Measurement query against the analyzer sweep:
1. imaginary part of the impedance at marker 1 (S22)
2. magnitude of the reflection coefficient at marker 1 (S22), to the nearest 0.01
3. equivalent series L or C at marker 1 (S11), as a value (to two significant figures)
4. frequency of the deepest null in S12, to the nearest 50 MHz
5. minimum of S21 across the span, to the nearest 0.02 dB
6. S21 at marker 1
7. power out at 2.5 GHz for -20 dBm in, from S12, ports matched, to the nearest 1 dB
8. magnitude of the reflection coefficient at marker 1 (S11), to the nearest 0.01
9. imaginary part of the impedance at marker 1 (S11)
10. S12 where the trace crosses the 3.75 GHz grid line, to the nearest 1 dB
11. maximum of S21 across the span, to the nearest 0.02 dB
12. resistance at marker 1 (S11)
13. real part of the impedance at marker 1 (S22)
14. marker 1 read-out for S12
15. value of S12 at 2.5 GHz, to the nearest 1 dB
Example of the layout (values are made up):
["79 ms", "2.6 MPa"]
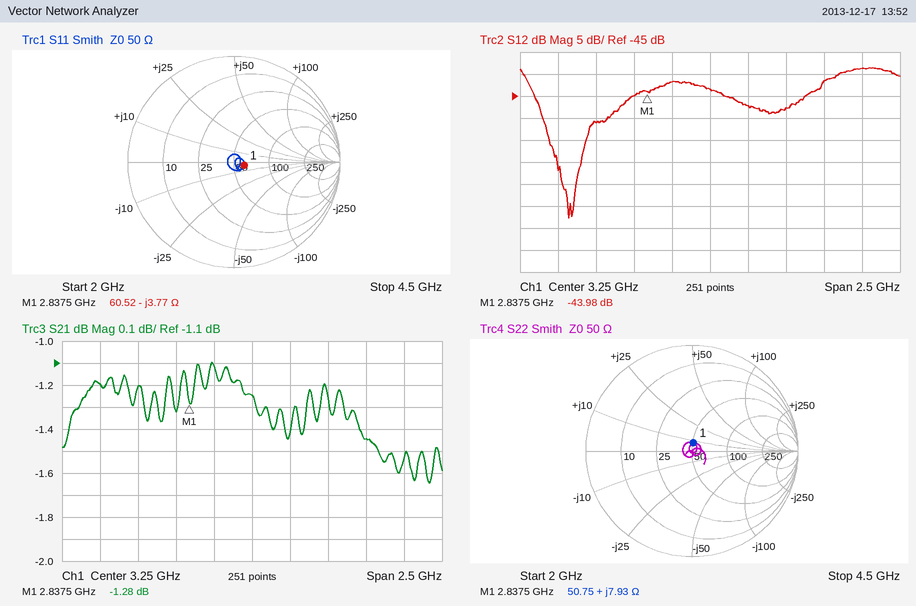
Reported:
["+7.93 Ω", "0.08", "15 pF", "2.30 GHz", "-1.64 dB", "-1.28 dB", "-71 dBm", "0.10", "-3.77 Ω", "-48 dB", "-1.10 dB", "60.52 Ω", "50.75 Ω", "-43.98 dB", "-51 dB"]
